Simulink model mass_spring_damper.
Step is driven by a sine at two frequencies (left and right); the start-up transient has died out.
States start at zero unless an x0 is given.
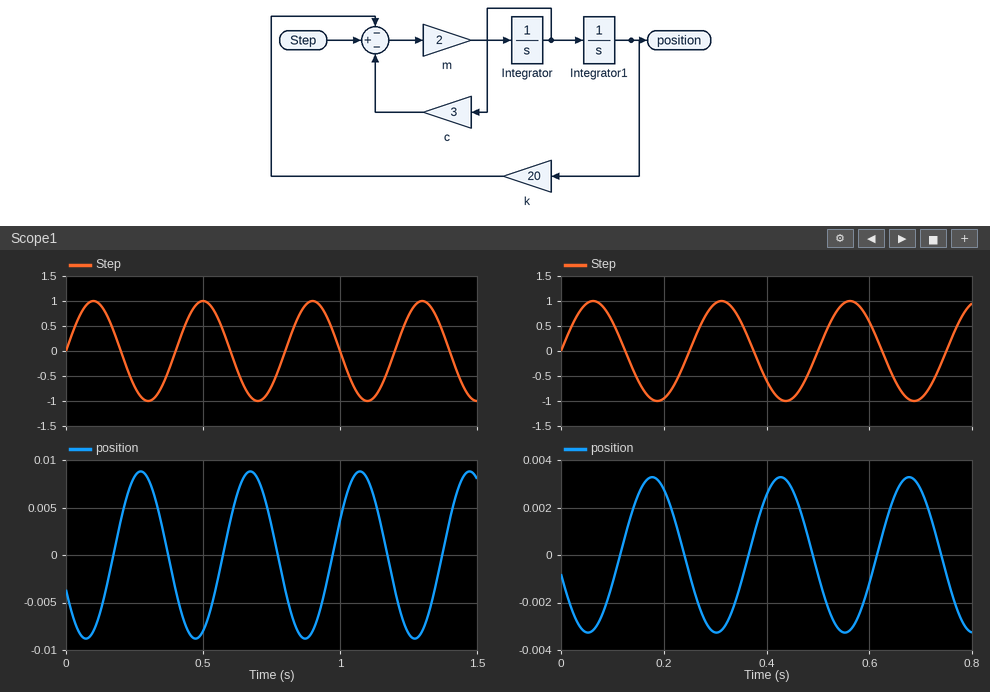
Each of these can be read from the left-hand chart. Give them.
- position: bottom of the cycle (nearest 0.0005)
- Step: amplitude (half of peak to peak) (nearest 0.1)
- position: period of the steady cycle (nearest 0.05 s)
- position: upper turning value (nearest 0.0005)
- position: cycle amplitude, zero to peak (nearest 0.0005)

-0.0090
1.0
0.40 s
0.0090
0.0090
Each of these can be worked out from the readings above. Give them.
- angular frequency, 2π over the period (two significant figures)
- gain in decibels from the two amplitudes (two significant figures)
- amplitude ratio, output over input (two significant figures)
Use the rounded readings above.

16 rad/s
-41 dB
0.0090
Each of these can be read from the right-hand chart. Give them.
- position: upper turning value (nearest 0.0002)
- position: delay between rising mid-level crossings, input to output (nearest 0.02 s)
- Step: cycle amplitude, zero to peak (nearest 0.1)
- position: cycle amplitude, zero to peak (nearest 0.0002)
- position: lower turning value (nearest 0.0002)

0.0032
0.12 s
1.0
0.0032
-0.0032
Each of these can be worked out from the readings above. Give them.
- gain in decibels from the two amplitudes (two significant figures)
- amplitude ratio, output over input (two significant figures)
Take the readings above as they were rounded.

-50 dB
0.0032
